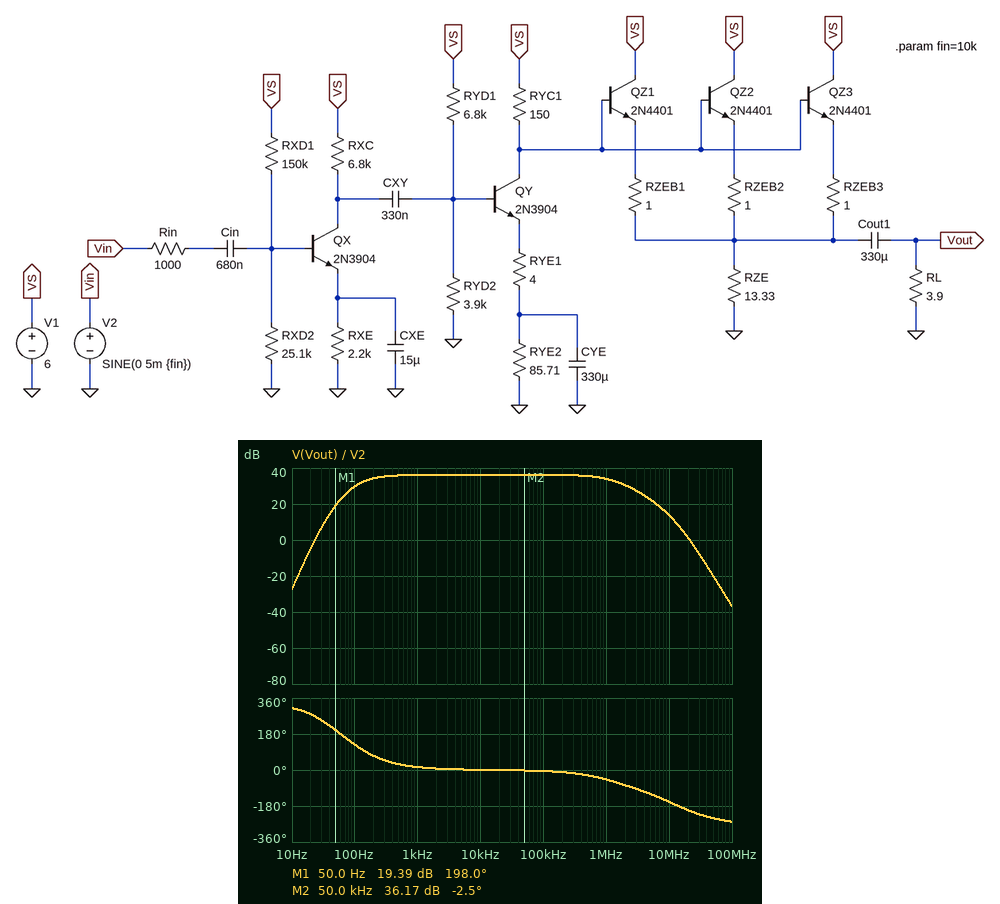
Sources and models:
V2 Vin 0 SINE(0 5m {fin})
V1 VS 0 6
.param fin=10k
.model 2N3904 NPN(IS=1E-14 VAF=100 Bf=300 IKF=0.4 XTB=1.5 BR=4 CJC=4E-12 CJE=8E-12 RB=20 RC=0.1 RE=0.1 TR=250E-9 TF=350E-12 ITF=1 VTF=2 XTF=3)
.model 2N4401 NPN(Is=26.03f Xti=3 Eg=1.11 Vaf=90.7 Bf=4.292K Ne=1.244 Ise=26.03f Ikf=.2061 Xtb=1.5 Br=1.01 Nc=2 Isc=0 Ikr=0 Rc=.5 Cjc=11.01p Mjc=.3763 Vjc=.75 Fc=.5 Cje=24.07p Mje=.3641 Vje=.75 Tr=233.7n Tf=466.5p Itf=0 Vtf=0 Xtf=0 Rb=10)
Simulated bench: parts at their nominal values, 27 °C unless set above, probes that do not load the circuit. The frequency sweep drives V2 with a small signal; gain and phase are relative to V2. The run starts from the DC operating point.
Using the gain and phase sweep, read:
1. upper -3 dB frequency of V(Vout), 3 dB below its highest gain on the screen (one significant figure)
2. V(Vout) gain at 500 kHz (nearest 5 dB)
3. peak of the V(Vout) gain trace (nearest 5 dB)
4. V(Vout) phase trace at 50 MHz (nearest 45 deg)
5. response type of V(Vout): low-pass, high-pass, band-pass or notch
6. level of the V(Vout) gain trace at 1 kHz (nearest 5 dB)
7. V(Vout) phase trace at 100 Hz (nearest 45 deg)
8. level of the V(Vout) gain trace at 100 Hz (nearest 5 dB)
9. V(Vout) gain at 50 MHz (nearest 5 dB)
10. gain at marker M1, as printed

1 MHz
35 dB
35 dB
-225 deg
band-pass
35 dB
135 deg
30 dB
-20 dB
19.39 dB
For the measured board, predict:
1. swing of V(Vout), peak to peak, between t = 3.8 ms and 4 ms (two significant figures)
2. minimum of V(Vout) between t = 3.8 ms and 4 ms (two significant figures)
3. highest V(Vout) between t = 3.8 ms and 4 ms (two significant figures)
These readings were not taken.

640 mV
-310 mV
330 mV
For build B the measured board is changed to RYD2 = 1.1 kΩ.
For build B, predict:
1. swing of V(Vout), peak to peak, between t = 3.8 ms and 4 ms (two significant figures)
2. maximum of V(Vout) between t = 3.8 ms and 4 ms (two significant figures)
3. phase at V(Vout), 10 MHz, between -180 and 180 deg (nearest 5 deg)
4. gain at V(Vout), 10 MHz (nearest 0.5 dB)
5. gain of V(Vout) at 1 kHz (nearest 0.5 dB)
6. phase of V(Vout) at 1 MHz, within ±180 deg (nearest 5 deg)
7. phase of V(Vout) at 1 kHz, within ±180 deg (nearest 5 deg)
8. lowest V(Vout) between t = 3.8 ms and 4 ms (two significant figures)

170 mV
80 mV
-150 deg
9.5 dB
24.5 dB
-25 deg
15 deg
-86 mV
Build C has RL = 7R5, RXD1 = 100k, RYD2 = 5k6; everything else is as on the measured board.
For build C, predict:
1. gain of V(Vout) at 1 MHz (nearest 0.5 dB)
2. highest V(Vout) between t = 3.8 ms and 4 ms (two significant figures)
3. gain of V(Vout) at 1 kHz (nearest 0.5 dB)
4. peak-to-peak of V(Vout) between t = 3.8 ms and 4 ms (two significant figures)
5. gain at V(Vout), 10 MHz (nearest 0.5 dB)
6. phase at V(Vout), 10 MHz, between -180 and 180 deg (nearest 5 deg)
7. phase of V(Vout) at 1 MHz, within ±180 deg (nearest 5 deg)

41.5 dB
870 mV
44.5 dB
1.6 V
20.5 dB
-155 deg
-55 deg
